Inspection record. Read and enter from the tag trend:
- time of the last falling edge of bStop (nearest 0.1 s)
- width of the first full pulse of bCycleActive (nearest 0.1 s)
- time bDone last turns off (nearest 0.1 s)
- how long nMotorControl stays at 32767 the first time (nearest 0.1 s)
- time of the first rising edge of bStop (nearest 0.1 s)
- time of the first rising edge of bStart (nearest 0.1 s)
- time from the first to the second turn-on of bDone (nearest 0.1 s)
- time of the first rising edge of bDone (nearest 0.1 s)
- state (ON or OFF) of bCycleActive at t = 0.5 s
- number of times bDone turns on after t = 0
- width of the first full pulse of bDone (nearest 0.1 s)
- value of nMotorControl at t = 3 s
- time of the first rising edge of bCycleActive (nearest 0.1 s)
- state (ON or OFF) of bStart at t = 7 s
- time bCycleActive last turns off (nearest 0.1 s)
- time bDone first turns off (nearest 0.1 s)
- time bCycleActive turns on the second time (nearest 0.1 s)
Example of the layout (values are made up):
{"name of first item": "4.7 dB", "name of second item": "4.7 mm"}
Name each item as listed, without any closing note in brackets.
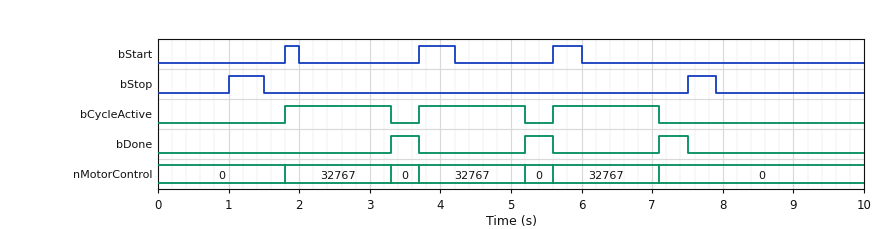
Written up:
{"time of the last falling edge of bStop": "7.9 s", "width of the first full pulse of bCycleActive": "1.5 s", "time bDone last turns off": "7.5 s", "how long nMotorControl stays at 32767 the first time": "1.5 s", "time of the first rising edge of bStop": "1.0 s", "time of the first rising edge of bStart": "1.8 s", "time from the first to the second turn-on of bDone": "1.9 s", "time of the first rising edge of bDone": "3.3 s", "state (ON or OFF) of bCycleActive at t = 0.5 s": "OFF", "number of times bDone turns on after t = 0": "3", "width of the first full pulse of bDone": "0.4 s", "value of nMotorControl at t = 3 s": "32767", "time of the first rising edge of bCycleActive": "1.8 s", "state (ON or OFF) of bStart at t = 7 s": "OFF", "time bCycleActive last turns off": "7.1 s", "time bDone first turns off": "3.7 s", "time bCycleActive turns on the second time": "3.7 s"}
